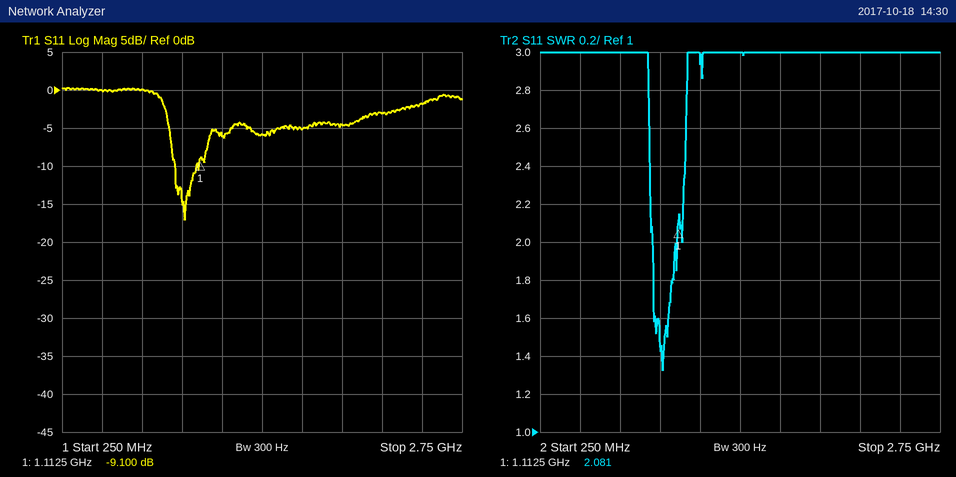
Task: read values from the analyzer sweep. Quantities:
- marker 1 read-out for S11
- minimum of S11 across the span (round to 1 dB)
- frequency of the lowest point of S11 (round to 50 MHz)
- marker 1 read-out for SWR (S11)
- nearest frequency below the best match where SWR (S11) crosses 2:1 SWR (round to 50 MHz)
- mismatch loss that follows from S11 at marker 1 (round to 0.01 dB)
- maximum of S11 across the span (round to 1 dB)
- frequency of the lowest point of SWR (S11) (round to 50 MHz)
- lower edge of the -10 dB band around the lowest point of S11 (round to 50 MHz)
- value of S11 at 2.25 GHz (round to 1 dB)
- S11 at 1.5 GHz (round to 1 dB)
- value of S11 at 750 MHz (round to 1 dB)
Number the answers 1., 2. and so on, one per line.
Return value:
1. -9.100 dB
2. -17 dB
3. 1.00 GHz
4. 2.081
5. 950 MHz
6. 0.57 dB
7. 0 dB
8. 1.00 GHz
9. 950 MHz
10. -3 dB
11. -6 dB
12. 0 dB
